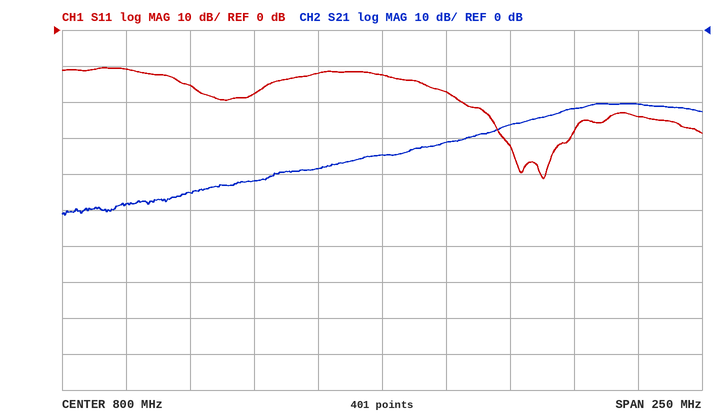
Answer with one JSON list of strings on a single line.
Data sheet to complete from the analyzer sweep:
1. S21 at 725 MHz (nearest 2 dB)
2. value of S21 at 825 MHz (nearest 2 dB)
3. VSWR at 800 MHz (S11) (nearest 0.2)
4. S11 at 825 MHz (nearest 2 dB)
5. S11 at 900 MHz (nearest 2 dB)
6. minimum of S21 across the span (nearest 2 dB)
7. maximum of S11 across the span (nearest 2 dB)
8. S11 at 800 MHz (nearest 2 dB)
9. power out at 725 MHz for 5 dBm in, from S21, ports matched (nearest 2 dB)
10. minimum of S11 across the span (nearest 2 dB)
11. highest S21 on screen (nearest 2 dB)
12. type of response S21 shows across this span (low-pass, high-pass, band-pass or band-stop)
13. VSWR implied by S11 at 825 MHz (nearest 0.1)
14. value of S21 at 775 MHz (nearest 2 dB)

["-46 dB", "-32 dB", "1.6", "-18 dB", "-24 dB", "-52 dB", "-10 dB", "-12 dB", "-40 dBm", "-42 dB", "-20 dB", "high-pass", "1.3", "-38 dB"]
